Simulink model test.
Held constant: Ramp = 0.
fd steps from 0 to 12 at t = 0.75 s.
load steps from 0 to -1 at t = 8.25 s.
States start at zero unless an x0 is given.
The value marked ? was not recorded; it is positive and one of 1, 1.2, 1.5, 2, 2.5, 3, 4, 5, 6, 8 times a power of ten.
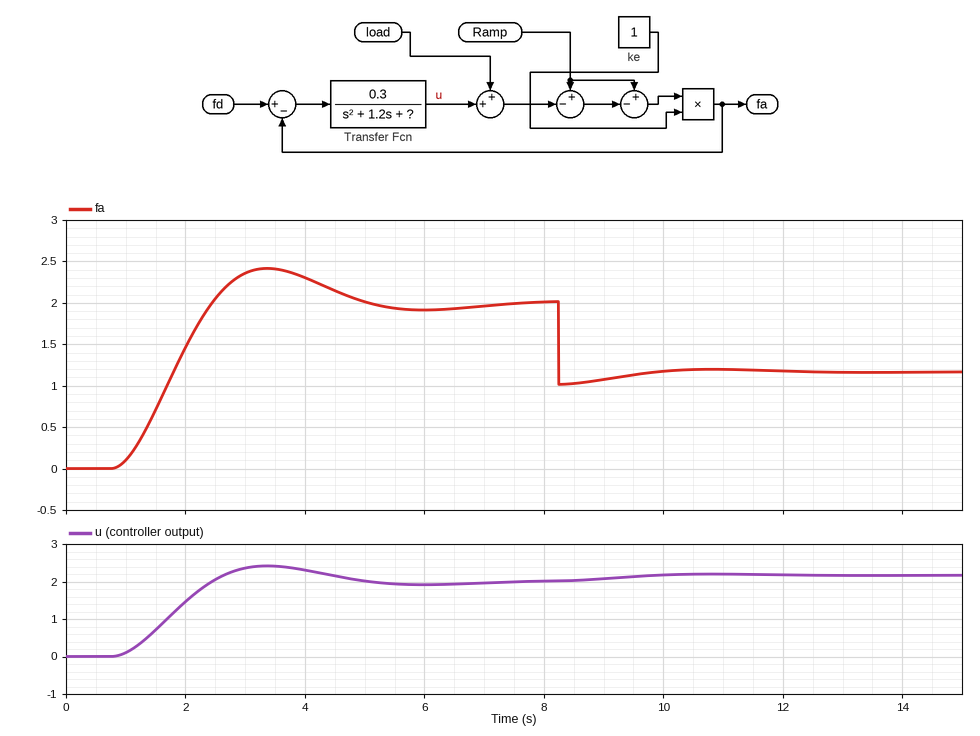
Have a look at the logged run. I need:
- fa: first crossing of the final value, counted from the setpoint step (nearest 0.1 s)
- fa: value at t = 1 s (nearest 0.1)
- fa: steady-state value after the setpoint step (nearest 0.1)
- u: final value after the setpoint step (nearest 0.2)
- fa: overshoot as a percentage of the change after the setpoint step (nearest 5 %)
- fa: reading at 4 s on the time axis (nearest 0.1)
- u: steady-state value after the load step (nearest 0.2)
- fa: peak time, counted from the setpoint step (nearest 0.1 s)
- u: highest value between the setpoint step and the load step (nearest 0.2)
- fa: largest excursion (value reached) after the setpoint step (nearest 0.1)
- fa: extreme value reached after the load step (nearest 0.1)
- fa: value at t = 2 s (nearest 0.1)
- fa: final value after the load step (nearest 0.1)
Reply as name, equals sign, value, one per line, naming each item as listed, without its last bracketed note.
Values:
fa: first crossing of the final value, counted from the setpoint step = 1.7 s
fa: value at t = 1 s = 0.1
fa: steady-state value after the setpoint step = 2.0
u: final value after the setpoint step = 2.0
fa: overshoot as a percentage of the change after the setpoint step = 20 %
fa: reading at 4 s on the time axis = 2.3
u: steady-state value after the load step = 2.2
fa: peak time, counted from the setpoint step = 2.6 s
u: highest value between the setpoint step and the load step = 2.4
fa: largest excursion (value reached) after the setpoint step = 2.4
fa: extreme value reached after the load step = 1.0
fa: value at t = 2 s = 1.5
fa: final value after the load step = 1.2
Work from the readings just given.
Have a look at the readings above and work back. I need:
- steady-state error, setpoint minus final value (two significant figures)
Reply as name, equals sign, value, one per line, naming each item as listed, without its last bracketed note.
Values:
steady-state error, setpoint minus final value = 10
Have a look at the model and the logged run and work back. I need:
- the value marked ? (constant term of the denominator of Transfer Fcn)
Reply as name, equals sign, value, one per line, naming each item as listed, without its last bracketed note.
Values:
the value marked ? = 1.5
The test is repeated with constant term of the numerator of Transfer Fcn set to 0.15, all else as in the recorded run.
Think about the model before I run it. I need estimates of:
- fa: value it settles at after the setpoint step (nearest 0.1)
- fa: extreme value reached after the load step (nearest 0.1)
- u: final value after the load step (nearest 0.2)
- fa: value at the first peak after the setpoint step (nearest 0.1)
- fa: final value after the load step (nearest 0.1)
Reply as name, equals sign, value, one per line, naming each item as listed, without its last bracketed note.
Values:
fa: value it settles at after the setpoint step = 1.1
fa: extreme value reached after the load step = 0.1
u: final value after the load step = 1.2
fa: value at the first peak after the setpoint step = 1.3
fa: final value after the load step = 0.2
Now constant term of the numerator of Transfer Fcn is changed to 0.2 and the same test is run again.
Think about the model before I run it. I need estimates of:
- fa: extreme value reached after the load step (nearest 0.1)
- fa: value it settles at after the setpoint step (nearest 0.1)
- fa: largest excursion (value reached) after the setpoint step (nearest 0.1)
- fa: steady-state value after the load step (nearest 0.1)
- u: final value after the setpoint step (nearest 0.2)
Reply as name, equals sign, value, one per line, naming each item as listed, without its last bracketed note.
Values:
fa: extreme value reached after the load step = 0.4
fa: value it settles at after the setpoint step = 1.4
fa: largest excursion (value reached) after the setpoint step = 1.7
fa: steady-state value after the load step = 0.5
u: final value after the setpoint step = 1.4
